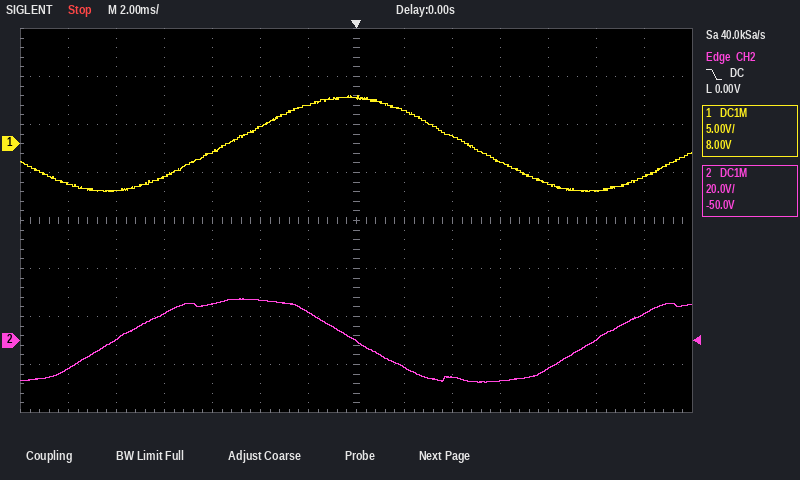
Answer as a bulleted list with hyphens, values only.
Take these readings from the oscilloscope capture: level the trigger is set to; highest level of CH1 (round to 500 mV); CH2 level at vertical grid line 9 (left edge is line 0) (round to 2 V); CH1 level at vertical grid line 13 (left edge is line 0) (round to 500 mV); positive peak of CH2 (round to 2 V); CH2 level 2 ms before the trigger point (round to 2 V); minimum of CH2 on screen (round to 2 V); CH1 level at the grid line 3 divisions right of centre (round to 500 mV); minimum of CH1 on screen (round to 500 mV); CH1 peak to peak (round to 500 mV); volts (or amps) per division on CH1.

- 0.00 V
- 5.0 V
- -16 V
- -3.5 V
- 18 V
- 12 V
- -18 V
- -2.0 V
- -5.0 V
- 10.0 V
- 5 V
